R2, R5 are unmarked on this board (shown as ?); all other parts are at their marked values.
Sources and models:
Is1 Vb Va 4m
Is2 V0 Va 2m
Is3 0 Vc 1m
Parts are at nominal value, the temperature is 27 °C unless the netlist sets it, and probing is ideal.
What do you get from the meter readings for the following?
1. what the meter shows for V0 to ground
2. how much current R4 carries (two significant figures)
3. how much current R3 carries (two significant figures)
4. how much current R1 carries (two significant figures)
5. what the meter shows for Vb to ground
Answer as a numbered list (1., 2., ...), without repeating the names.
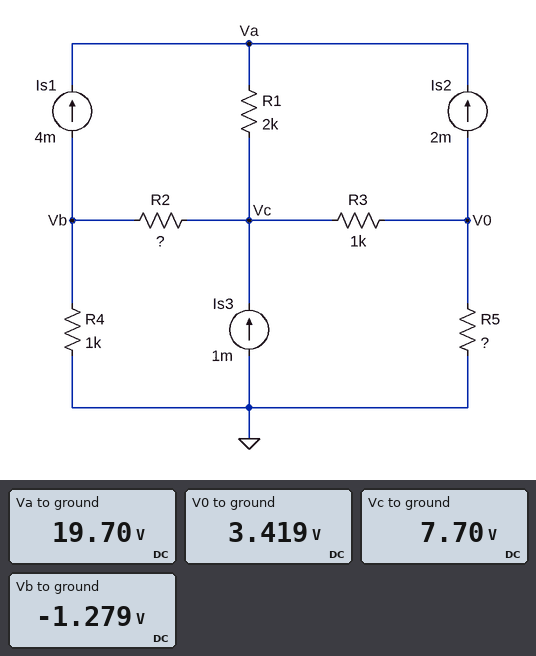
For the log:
1. 3.419 V
2. 1.3 mA
3. 4.3 mA
4. 6.0 mA
5. -1.279 V
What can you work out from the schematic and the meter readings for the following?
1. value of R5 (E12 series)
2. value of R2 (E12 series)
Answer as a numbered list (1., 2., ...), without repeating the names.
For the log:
1. 1.5 kΩ
2. 3.3 kΩ
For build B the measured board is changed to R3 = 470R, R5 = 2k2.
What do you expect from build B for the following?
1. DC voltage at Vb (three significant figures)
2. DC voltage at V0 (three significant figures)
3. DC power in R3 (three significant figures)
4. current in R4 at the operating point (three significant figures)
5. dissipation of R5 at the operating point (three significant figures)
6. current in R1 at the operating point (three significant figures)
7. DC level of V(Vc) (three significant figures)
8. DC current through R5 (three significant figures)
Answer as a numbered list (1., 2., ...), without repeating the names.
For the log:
1. -1.38 V
2. 5.23 V
3. 9.00 mW
4. 1.38 mA
5. 12.4 mW
6. 6.00 mA
7. 7.28 V
8. 2.38 mA
